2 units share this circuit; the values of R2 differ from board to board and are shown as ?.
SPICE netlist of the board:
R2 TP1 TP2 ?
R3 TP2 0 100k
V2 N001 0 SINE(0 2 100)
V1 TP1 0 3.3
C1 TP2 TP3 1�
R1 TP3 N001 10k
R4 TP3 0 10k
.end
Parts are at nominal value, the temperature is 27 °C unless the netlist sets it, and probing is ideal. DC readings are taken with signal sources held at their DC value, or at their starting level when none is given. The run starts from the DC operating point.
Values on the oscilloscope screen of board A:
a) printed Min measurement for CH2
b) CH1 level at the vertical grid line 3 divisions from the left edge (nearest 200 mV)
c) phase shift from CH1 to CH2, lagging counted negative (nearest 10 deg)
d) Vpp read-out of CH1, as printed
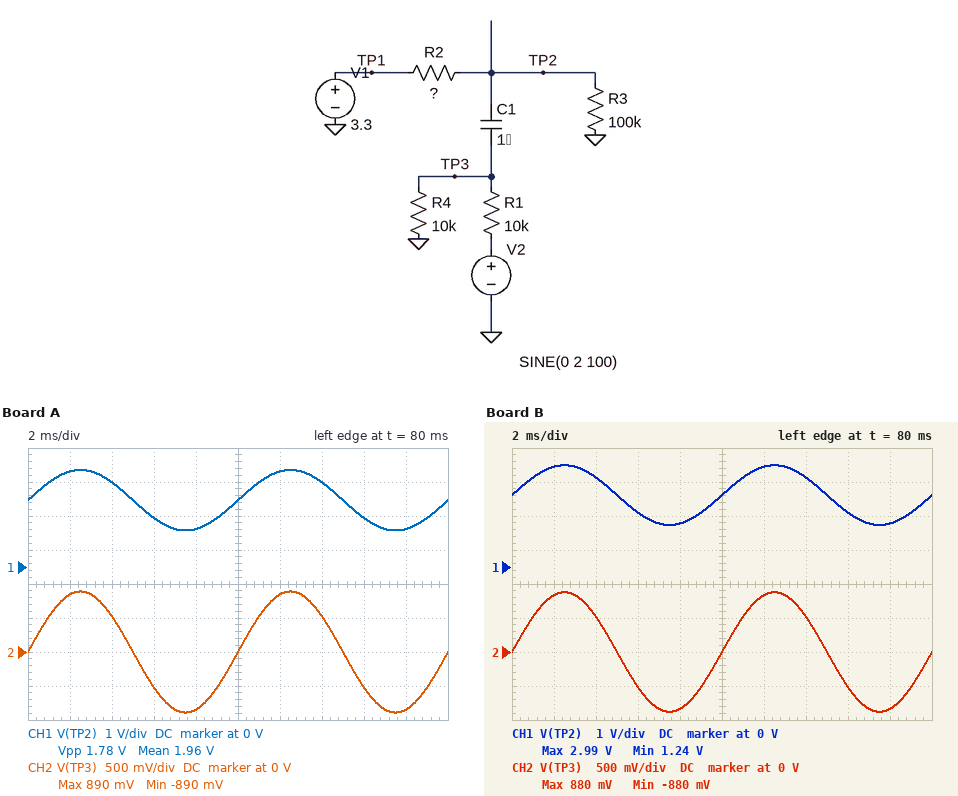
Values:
-890 mV
1.4 V
0 deg
1.78 V
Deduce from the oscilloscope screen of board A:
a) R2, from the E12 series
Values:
68 kΩ
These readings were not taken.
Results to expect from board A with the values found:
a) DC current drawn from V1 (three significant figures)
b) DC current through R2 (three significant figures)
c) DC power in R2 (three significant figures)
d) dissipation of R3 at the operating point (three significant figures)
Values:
19.6 µA
19.6 µA
26.2 µW
38.6 µW
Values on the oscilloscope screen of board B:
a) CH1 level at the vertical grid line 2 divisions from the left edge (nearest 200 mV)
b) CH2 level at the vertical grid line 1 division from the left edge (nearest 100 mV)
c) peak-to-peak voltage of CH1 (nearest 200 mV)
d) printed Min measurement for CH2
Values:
2.6 V
800 mV
1.8 V
-880 mV
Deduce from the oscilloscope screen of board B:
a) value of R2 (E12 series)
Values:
56 kΩ
